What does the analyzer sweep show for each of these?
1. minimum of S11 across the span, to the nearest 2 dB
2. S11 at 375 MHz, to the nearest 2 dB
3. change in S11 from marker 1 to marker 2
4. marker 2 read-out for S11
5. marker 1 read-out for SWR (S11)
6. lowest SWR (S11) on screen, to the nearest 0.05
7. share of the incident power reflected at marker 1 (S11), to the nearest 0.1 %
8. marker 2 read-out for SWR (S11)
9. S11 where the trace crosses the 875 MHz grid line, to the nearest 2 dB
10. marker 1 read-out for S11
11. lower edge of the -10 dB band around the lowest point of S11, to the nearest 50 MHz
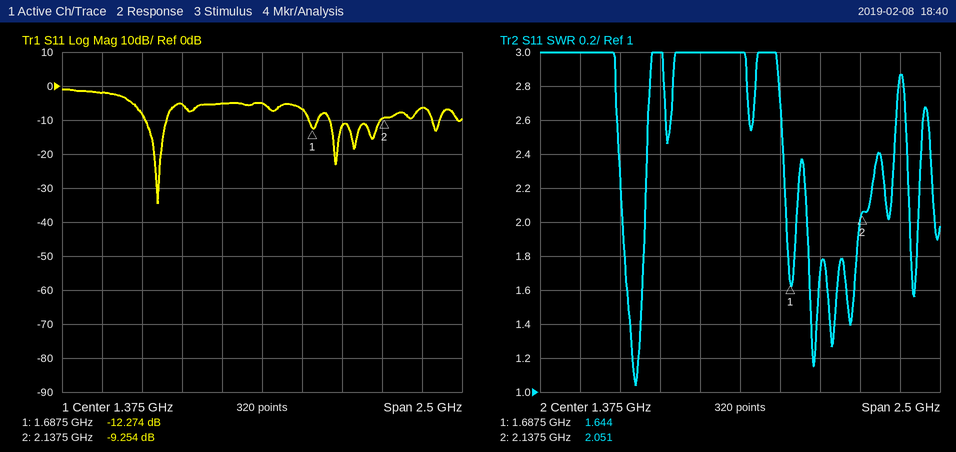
-34 dB
-2 dB
3.020 dB
-9.254 dB
1.644
1.05
5.9 %
2.051
-6 dB
-12.274 dB
650 MHz
